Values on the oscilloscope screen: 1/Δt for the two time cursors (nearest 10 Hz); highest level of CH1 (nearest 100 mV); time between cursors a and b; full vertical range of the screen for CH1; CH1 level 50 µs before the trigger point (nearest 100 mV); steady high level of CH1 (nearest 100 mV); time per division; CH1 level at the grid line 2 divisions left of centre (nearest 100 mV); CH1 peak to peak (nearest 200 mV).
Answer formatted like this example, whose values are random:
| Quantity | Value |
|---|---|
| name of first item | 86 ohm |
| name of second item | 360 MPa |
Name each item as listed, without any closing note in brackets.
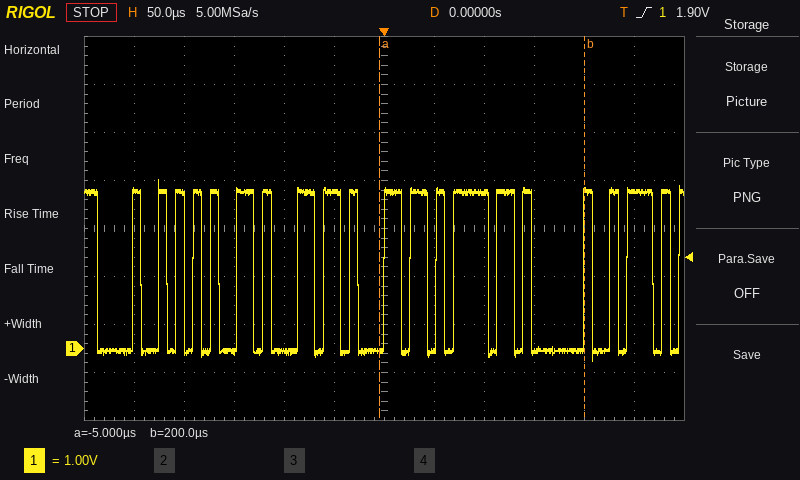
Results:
| Quantity | Value |
|---|---|
| 1/Δt for the two time cursors | 4.88 kHz |
| highest level of CH1 | 3.5 V |
| time between cursors a and b | 205 µs |
| full vertical range of the screen for CH1 | 8 V |
| CH1 level 50 µs before the trigger point | 3.3 V |
| steady high level of CH1 | 3.3 V |
| time per division | 50 µs |
| CH1 level at the grid line 2 divisions left of centre | -100 mV |
| CH1 peak to peak | 3.8 V |
